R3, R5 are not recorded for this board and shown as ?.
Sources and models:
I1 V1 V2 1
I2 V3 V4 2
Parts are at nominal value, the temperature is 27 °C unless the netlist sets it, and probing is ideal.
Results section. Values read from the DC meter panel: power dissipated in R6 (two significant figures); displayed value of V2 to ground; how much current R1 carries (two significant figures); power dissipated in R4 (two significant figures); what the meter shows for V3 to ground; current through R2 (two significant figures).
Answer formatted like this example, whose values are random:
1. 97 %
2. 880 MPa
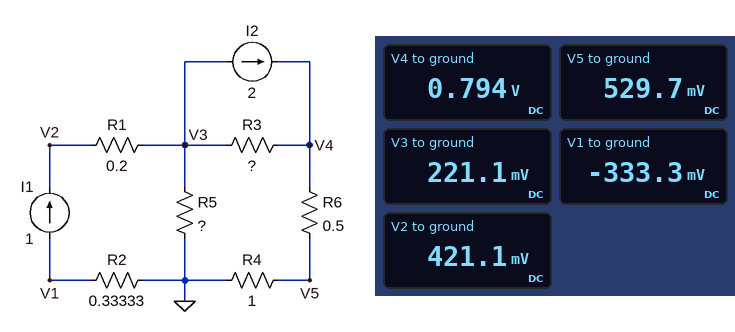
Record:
1. 140 mW
2. 421.1 mV
3. 1.0 A
4. 280 mW
5. 221.1 mV
6. 1.0 A
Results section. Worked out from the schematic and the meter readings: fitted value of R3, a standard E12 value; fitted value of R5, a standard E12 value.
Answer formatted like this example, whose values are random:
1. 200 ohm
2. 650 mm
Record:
1. 0.39 Ω
2. 0.47 Ω
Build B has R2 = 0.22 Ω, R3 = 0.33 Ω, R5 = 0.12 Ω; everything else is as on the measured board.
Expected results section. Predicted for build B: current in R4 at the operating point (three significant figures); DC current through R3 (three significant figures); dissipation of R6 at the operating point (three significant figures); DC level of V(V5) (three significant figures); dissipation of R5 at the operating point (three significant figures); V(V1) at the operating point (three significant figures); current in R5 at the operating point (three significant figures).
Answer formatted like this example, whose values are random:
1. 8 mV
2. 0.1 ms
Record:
1. 400 mA
2. 1.60 A
3. 80.0 mW
4. 400 mV
5. 43.2 mW
6. -220 mV
7. 600 mA
